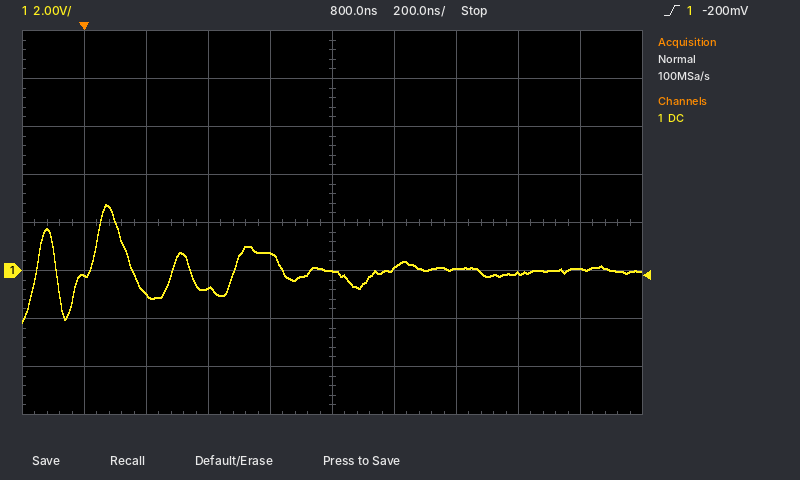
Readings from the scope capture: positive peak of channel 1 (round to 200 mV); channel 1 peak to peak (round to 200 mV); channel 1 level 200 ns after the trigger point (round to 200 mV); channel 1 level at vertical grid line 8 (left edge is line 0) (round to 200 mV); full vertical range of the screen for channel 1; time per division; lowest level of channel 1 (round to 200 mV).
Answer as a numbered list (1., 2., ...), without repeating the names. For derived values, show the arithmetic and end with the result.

1. 2.8 V
2. 2.8 V − (-2.2 V) = 5.0 V
3. -1.0 V
4. -200 mV
5. 16 V
6. 200 ns
7. -2.2 V
